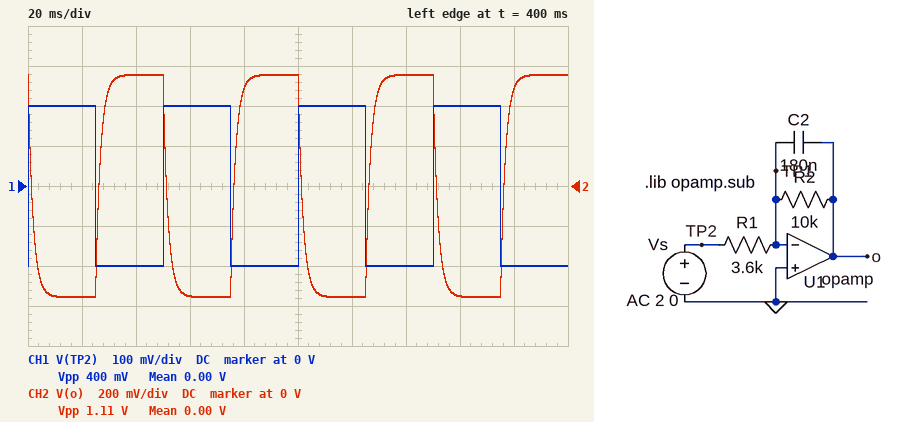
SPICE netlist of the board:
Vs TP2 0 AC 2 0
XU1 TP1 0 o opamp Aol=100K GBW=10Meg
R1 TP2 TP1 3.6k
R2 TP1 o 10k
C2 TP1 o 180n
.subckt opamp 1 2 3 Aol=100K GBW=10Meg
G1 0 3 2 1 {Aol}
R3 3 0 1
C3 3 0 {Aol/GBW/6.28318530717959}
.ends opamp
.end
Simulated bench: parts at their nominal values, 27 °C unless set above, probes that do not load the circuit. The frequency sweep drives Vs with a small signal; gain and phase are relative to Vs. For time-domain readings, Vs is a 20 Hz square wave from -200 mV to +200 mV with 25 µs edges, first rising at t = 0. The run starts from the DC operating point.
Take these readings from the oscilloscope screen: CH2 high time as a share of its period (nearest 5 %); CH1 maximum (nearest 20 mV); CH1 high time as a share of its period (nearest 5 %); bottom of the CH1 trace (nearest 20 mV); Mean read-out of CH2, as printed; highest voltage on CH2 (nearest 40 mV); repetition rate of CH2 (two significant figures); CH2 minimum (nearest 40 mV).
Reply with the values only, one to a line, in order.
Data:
50 %
200 mV
50 %
-200 mV
0.00 V
560 mV
20 Hz
-560 mV
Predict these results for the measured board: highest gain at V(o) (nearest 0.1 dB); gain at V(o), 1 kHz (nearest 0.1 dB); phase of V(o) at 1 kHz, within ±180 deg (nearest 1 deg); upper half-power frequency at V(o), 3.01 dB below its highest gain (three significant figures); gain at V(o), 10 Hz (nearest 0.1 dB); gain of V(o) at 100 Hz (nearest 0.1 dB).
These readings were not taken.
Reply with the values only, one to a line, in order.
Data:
8.9 dB
-12.2 dB
95 deg
88.4 Hz
8.8 dB
5.3 dB
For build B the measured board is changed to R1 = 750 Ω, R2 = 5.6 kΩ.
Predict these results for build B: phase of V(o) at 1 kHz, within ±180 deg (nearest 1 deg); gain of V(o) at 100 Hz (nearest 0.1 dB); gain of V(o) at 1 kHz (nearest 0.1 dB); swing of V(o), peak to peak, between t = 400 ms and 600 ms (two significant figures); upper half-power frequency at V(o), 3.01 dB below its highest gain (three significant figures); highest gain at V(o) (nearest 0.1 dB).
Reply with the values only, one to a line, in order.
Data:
99 deg
16.0 dB
1.3 dB
3.0 V
158 Hz
17.5 dB
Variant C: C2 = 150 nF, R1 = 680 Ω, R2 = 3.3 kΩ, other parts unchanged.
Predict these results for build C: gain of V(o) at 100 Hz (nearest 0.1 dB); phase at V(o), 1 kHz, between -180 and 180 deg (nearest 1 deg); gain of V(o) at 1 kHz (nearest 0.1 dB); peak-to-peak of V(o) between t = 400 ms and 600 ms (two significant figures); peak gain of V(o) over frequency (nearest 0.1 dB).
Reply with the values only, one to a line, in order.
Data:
13.3 dB
108 deg
3.4 dB
1.9 V
13.7 dB
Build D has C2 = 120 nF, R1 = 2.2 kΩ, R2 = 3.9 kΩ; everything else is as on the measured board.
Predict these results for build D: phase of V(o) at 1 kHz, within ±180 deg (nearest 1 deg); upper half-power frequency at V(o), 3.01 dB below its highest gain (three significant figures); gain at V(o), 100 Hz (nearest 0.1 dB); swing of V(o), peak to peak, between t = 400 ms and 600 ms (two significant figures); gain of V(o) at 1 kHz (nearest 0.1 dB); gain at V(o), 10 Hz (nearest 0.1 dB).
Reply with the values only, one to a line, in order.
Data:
109 deg
340 Hz
4.6 dB
710 mV
-4.9 dB
5.0 dB
